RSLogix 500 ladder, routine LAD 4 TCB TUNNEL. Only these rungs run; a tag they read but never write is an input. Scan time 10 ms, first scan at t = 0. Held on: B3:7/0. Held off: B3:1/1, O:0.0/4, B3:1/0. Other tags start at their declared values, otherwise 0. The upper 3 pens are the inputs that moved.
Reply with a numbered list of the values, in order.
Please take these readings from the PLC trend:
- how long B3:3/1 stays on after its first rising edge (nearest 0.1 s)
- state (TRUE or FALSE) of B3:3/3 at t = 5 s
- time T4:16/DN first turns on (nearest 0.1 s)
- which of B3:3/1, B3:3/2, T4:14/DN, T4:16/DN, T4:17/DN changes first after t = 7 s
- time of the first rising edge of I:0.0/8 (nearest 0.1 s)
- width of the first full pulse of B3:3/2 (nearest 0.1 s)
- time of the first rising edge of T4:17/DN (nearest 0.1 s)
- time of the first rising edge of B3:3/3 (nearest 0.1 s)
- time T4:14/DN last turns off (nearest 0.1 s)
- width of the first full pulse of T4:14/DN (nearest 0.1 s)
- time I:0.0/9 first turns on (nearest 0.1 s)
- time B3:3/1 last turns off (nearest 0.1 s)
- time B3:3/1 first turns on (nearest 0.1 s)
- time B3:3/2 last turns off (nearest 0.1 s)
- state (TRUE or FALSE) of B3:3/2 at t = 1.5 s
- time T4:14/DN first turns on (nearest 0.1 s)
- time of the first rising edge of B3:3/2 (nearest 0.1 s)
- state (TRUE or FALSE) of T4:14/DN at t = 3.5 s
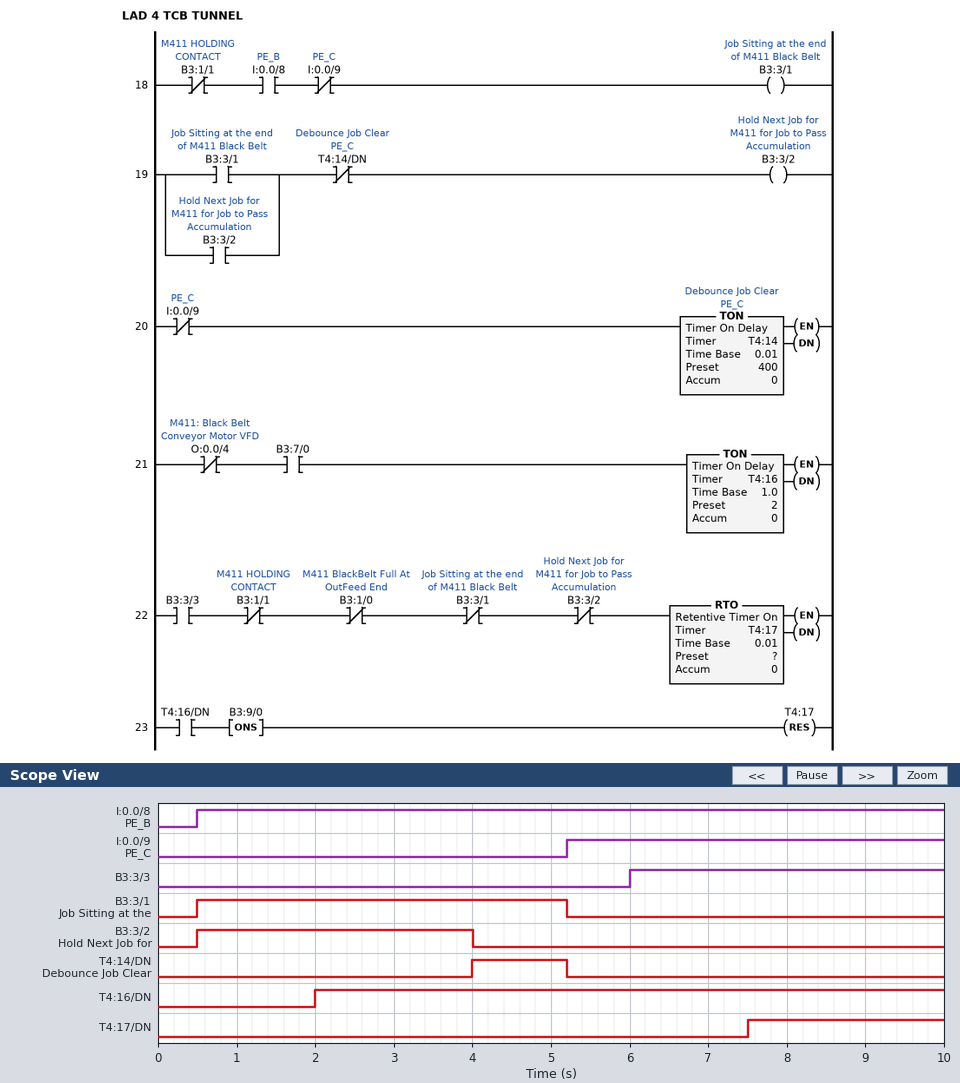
1. 4.7 s
2. FALSE
3. 2.0 s
4. T4:17/DN
5. 0.5 s
6. 3.5 s
7. 7.5 s
8. 6.0 s
9. 5.2 s
10. 1.2 s
11. 5.2 s
12. 5.2 s
13. 0.5 s
14. 4.0 s
15. TRUE
16. 4.0 s
17. 0.5 s
18. FALSE
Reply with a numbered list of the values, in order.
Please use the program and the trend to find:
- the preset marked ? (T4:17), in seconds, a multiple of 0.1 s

1. 1.5 s
